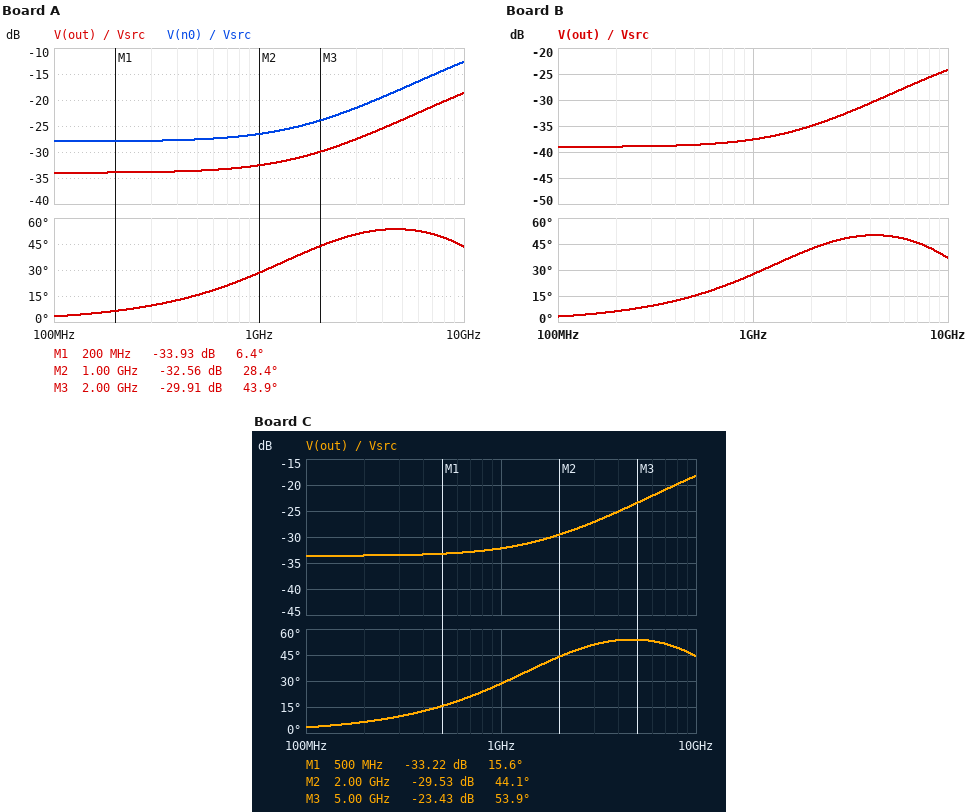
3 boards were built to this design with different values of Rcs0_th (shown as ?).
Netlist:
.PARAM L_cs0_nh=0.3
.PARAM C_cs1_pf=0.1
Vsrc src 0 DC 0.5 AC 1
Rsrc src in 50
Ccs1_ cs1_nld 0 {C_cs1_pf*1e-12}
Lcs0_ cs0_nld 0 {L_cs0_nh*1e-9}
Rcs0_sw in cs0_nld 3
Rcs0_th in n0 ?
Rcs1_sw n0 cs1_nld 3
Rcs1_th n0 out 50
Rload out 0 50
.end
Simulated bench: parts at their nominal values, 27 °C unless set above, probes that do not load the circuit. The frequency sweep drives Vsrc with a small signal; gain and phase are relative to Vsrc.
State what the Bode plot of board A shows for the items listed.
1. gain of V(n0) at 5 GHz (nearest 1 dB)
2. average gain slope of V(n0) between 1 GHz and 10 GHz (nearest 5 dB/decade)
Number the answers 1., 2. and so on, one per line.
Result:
1. -18 dB
2. 15 dB/decade
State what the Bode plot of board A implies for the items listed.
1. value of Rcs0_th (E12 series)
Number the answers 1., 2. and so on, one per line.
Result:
1. 39 Ω
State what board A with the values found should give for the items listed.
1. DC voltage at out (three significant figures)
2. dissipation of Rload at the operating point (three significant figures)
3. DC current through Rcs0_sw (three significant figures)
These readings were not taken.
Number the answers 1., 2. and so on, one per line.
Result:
1. 9.98 mV
2. 1.99 µW
3. 9.25 mA
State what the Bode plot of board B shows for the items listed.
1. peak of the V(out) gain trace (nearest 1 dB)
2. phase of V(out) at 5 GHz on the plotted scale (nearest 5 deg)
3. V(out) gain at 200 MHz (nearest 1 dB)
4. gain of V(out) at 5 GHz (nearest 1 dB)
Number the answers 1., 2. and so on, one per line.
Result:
1. -24 dB
2. 50 deg
3. -39 dB
4. -29 dB
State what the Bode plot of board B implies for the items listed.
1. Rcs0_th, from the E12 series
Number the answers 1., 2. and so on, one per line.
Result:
1. 150 Ω
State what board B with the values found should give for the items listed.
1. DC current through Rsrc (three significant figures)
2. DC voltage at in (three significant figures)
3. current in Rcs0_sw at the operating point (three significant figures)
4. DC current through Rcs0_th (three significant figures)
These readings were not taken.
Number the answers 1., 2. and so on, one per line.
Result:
1. 9.44 mA
2. 28.0 mV
3. 9.33 mA
4. 112 µA
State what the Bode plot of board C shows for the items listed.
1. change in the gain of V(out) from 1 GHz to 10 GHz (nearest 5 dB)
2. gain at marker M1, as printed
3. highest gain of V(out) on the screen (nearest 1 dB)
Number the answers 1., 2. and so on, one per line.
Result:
1. 15 dB
2. -33.22 dB
3. -18 dB
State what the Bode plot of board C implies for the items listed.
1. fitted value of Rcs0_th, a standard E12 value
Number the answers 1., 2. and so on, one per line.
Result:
1. 33 Ω
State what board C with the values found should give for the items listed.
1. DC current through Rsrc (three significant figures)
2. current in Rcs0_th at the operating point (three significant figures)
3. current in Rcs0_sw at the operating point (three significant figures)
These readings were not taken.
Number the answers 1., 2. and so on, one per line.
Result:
1. 9.45 mA
2. 208 µA
3. 9.24 mA
